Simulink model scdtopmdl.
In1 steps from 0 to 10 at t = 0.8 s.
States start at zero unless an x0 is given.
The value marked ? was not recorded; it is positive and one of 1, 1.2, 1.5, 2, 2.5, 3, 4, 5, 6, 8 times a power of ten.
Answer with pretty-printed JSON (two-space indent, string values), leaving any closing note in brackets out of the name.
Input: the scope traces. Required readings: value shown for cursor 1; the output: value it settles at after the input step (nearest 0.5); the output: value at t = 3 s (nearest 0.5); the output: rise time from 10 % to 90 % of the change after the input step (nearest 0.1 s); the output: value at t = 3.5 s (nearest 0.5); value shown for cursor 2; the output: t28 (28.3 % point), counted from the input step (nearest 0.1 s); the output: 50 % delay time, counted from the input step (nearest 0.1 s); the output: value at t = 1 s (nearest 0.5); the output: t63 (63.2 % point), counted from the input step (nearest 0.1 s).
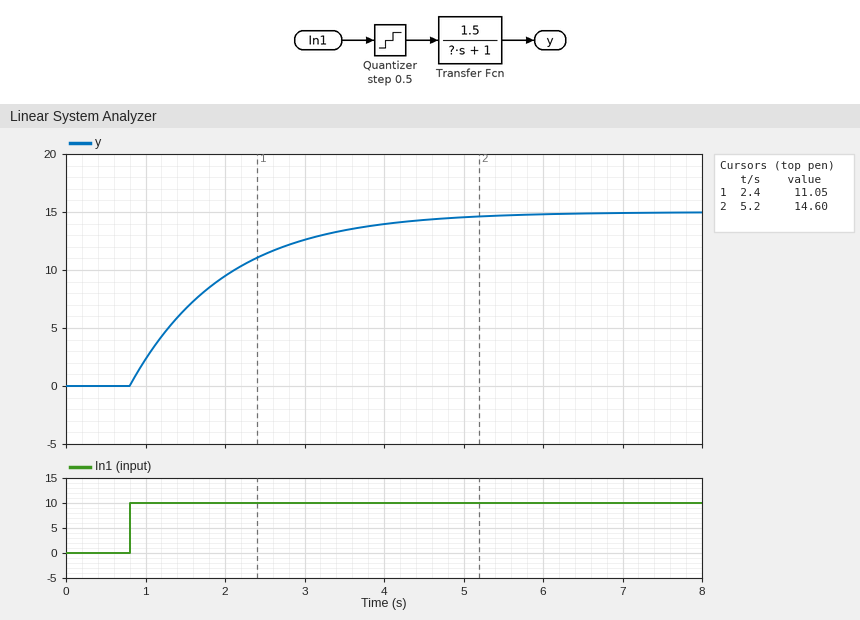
{
  "value shown for cursor 1": "11.05",
  "the output: value it settles at after the input step": "15.0",
  "the output: value at t = 3 s": "12.5",
  "the output: rise time from 10 % to 90 % of the change after the input step": "2.6 s",
  "the output: value at t = 3.5 s": "13.5",
  "value shown for cursor 2": "14.60",
  "the output: t28 (28.3 % point), counted from the input step": "0.4 s",
  "the output: 50 % delay time, counted from the input step": "0.8 s",
  "the output: value at t = 1 s": "2.5",
  "the output: t63 (63.2 % point), counted from the input step": "1.2 s"
}
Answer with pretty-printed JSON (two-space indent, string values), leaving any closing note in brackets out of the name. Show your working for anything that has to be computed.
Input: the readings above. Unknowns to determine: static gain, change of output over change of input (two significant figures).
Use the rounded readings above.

{
  "static gain, change of output over change of input": "(15 - 0) / (10 - 0) = 1.5"
}
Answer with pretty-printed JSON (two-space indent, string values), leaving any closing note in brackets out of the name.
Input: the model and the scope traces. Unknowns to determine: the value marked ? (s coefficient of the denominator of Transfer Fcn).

{
  "the value marked ?": "1.2"
}
